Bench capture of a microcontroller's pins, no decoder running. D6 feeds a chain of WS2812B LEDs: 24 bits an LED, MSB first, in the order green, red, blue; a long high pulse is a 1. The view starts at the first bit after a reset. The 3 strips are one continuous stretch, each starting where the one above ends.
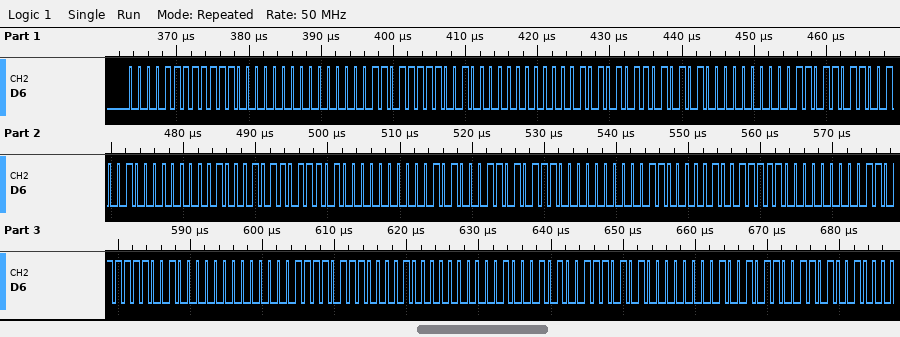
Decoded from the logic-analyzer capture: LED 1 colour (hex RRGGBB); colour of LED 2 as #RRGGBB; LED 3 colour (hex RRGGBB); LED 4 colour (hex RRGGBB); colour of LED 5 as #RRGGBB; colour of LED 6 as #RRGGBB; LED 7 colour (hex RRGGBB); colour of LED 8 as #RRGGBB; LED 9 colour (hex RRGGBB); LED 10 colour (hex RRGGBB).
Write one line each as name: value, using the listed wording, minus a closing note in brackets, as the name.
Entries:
LED 1 colour: #F00F00
colour of LED 2 as #RRGGBB: #E41B00
LED 3 colour: #D52A00
LED 4 colour: #C93600
colour of LED 5 as #RRGGBB: #BA4500
colour of LED 6 as #RRGGBB: #AE5100
LED 7 colour: #9F6000
colour of LED 8 as #RRGGBB: #906F00
LED 9 colour: #847B00
LED 10 colour: #758A00
